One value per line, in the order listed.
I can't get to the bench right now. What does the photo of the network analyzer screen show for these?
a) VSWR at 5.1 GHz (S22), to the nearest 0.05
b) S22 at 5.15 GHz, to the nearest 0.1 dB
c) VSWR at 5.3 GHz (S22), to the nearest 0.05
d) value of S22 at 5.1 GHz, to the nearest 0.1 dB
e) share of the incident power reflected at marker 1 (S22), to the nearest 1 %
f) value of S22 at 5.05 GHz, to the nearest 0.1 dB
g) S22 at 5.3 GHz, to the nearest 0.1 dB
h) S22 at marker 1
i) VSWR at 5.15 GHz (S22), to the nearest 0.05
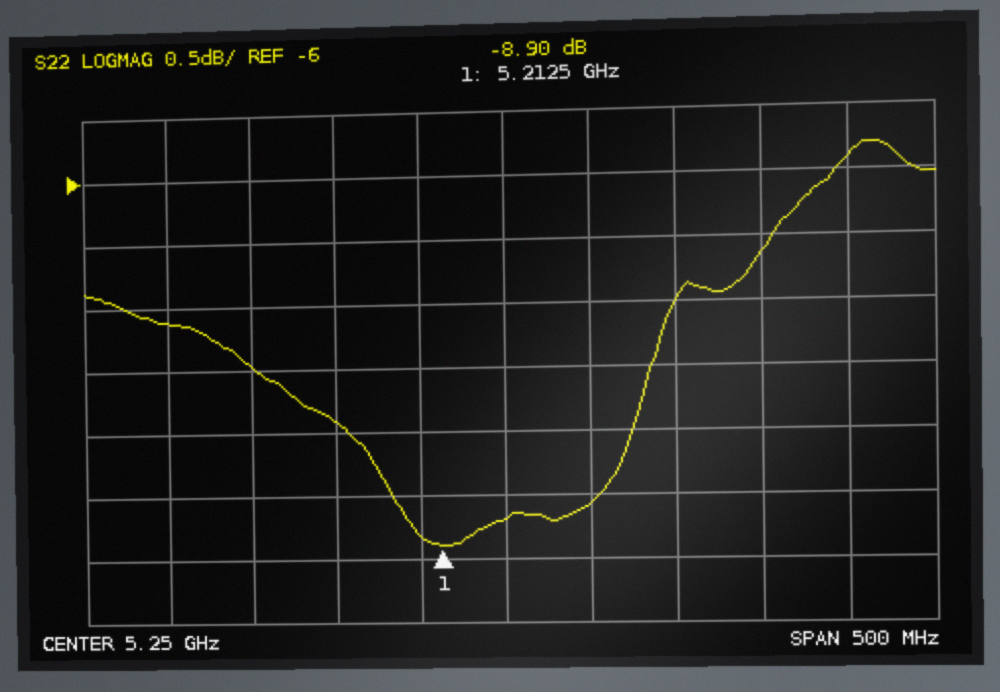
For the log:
2.45
-7.9 dB
2.20
-7.5 dB
13 %
-7.1 dB
-8.6 dB
-8.90 dB
2.35
